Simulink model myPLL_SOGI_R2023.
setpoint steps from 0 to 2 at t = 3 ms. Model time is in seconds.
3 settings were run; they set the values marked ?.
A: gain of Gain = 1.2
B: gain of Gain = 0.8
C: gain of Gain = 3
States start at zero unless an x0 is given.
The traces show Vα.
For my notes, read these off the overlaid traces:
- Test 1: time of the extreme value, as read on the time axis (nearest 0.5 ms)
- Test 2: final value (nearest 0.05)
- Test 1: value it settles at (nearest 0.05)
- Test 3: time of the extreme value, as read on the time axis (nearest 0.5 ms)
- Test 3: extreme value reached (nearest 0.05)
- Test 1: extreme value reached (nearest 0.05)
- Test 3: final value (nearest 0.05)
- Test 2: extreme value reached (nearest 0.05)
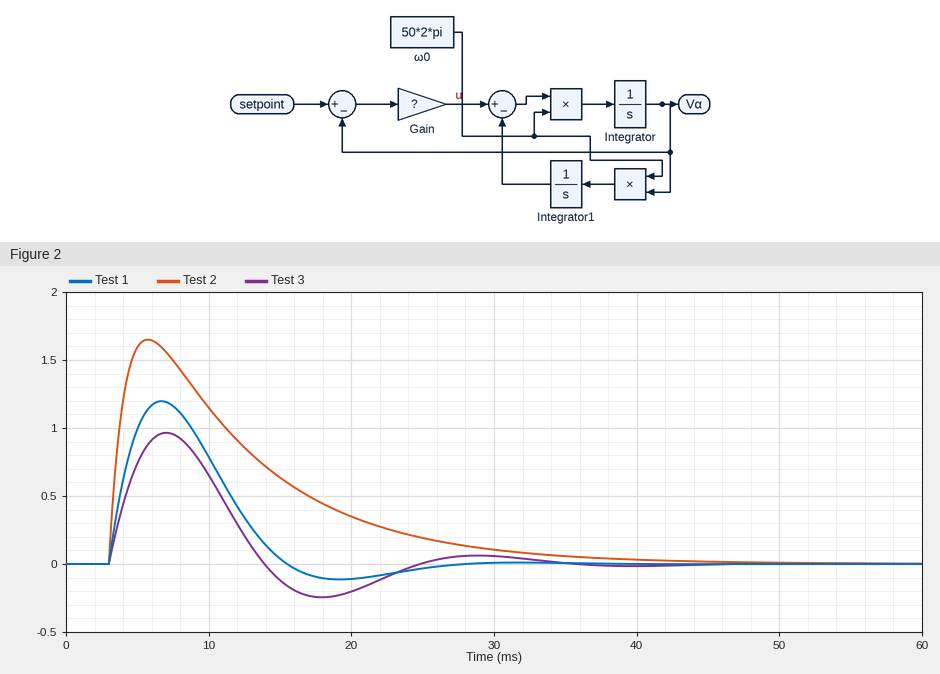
6.5 ms
0.00
0.00
7.0 ms
0.95
1.20
0.00
1.65
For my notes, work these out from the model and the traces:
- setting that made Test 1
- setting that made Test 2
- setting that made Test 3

A
C
B
